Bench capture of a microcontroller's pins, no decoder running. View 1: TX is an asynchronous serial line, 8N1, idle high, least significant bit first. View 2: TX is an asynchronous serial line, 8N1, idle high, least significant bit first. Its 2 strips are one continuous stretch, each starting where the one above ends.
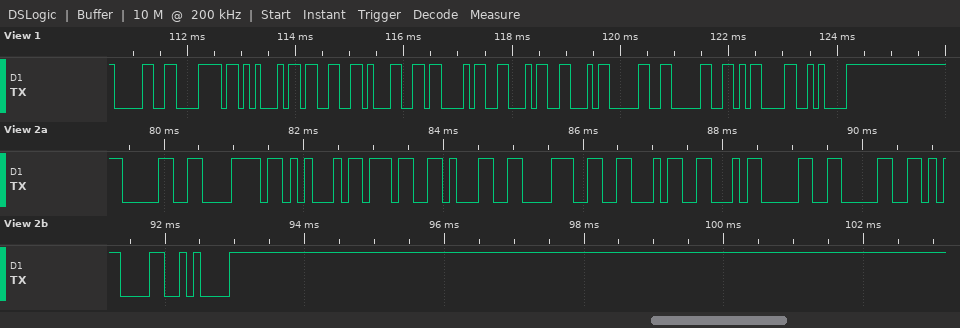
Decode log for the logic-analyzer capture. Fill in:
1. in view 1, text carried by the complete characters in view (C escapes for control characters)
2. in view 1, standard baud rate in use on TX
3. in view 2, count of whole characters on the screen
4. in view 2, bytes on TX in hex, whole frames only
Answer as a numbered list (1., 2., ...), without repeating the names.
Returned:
1. "0xE31CFF00\r\n"
2. 9600 baud
3. 12
4. 30 78 45 37 31 38 46 46 30 30 0D 0A
